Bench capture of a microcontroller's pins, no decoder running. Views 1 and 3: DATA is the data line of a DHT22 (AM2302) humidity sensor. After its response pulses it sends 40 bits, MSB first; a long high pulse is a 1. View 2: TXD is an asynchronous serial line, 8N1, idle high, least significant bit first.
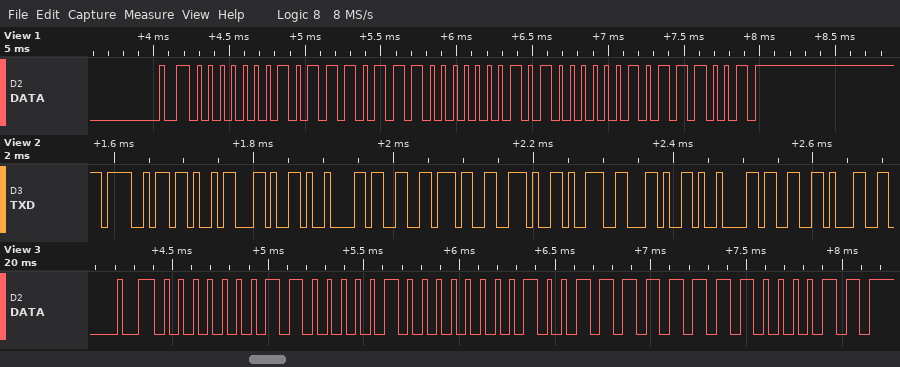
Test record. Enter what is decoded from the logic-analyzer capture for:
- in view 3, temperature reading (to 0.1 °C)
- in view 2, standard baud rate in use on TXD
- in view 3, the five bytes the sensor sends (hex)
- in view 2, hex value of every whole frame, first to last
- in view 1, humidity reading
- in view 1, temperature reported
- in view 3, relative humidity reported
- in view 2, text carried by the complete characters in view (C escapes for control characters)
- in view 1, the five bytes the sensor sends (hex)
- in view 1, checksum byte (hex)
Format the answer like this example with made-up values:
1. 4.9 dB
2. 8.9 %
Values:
1. 31.9 °C
2. 115200 baud
3. 01 82 01 3F C3
4. 4F 4B 2C 09 33 37 2E 39 2C 09 33 31
5. 37.5 %
6. 32.0 °C
7. 38.6 %
8. "OK,\t37.9,\t31"
9. 01 77 01 40 B9
10. 0xB9
